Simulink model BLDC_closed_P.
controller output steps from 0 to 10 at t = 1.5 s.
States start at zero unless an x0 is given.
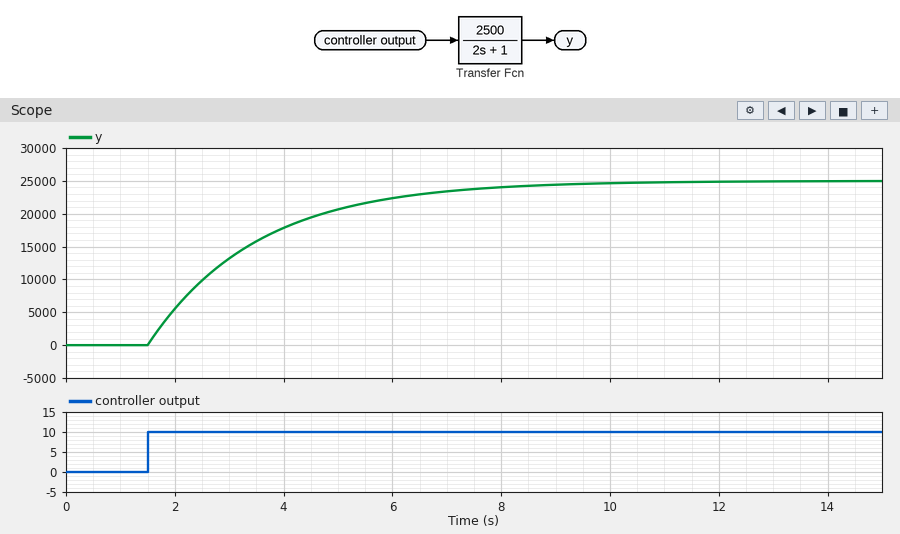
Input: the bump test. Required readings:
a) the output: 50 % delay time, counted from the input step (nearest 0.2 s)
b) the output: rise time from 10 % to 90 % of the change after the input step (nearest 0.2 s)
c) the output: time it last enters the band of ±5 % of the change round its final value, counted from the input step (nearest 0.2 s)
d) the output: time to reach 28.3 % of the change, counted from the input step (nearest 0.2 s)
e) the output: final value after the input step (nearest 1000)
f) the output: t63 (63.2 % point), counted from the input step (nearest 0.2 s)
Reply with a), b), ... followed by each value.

a) 1.4 s
b) 4.4 s
c) 6.0 s
d) 0.6 s
e) 25000
f) 2.0 s
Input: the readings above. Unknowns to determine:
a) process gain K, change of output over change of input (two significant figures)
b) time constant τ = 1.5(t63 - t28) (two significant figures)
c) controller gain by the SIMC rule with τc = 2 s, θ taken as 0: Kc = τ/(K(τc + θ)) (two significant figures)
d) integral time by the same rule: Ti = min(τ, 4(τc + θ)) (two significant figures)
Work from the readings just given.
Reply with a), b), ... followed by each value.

a) 2500
b) 2.1 s
c) 0.00042
d) 2.1 s
